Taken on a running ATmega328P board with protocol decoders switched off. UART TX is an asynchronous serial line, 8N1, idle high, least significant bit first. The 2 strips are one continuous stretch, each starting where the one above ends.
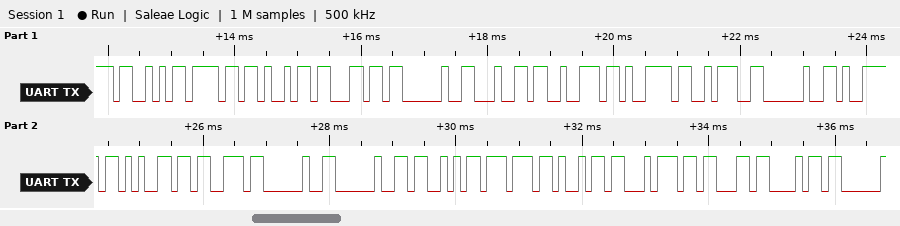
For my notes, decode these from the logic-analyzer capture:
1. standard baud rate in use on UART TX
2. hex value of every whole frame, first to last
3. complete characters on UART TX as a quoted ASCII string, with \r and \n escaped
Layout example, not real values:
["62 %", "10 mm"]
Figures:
["9600 baud", "53 6F 69 6C 20 64 72 79 3A 20 79 65 73 20 20 53 77 69 74 63 68", "\"Soil dry: yes  Switch\""]
